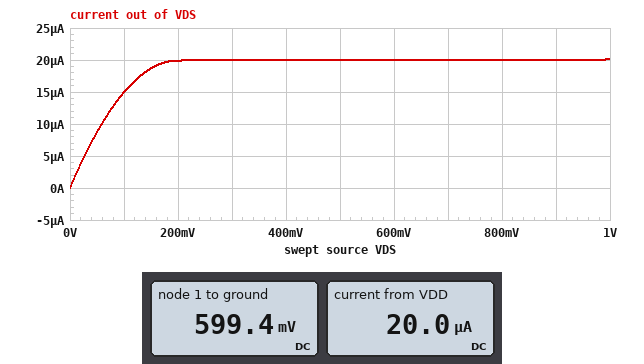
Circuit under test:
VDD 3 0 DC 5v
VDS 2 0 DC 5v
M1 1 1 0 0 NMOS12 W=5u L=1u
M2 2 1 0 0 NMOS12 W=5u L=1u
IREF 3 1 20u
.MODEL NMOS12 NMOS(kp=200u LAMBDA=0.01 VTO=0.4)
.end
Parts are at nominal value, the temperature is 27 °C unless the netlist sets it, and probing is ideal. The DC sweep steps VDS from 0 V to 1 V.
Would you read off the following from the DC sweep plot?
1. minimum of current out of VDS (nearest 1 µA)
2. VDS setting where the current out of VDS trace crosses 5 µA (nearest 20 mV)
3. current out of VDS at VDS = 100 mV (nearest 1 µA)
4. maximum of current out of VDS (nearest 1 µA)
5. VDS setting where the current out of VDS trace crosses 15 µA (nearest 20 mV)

0 A
20 mV
15 µA
20 µA
100 mV
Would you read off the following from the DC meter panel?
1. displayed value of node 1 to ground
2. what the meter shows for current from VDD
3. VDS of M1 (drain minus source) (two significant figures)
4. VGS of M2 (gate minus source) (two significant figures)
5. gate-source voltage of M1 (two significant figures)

599.4 mV
20.0 µA
600 mV
600 mV
600 mV
